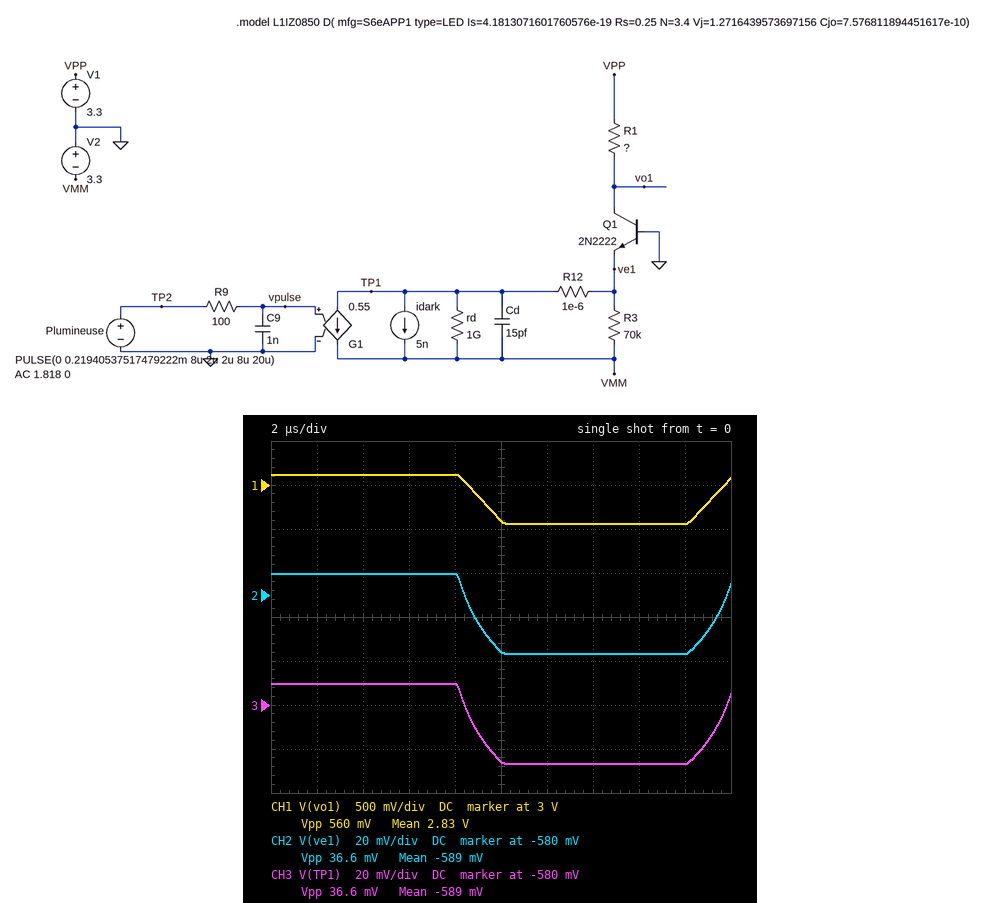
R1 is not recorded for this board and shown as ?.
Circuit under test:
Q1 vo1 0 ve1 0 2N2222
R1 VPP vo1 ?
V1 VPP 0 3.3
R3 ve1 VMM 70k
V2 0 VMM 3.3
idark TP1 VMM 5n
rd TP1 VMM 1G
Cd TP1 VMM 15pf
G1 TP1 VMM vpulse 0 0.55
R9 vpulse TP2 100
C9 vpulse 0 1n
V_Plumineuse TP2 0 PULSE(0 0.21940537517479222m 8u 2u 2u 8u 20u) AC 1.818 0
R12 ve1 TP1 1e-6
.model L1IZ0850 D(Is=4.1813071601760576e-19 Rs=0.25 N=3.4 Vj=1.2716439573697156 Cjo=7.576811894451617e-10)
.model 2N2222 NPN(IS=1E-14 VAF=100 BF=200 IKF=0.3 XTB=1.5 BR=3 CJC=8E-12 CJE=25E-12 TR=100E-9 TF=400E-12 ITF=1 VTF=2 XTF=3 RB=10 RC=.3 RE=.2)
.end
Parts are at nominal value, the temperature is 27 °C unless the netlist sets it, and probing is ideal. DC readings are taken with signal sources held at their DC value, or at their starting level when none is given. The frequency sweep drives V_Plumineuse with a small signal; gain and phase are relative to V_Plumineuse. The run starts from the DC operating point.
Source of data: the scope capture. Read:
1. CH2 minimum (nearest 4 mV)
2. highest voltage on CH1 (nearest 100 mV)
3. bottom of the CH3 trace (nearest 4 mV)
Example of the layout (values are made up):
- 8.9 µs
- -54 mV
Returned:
- -608 mV
- 3.1 V
- -608 mV
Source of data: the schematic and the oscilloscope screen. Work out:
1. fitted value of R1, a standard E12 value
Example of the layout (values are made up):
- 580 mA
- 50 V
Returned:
- 4.7 kΩ
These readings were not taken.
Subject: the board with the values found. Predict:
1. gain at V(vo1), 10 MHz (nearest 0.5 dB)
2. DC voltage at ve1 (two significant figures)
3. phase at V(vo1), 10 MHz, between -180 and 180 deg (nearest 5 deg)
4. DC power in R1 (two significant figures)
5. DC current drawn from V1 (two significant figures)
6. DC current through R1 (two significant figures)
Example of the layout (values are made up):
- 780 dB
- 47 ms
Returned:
- 40.0 dB
- -570 mV
- -20 deg
- 7.1 µW
- 39 µA
- 39 µA
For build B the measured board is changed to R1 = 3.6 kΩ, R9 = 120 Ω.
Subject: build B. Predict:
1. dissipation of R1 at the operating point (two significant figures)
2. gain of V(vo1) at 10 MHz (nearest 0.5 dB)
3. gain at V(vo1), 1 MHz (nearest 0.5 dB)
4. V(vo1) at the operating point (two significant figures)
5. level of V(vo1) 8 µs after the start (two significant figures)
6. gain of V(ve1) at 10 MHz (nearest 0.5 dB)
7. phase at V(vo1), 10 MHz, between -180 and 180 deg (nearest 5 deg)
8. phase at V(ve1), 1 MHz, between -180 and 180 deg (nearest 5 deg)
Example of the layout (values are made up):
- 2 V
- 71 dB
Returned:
- 5.4 µW
- 37.5 dB
- 63.5 dB
- 3.2 V
- 3.2 V
- 26.0 dB
- -15 deg
- 130 deg
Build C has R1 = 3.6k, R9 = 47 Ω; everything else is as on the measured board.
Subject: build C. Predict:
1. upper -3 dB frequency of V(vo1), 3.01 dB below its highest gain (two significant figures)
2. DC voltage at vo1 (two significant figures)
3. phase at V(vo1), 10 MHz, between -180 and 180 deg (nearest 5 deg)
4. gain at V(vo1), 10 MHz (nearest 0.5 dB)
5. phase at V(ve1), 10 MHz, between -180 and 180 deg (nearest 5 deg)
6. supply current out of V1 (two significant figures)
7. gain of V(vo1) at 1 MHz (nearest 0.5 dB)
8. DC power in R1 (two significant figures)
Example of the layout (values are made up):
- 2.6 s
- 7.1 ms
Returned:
- 2.4 MHz
- 3.2 V
- -5 deg
- 45.0 dB
- 45 deg
- 39 µA
- 65.0 dB
- 5.4 µW
